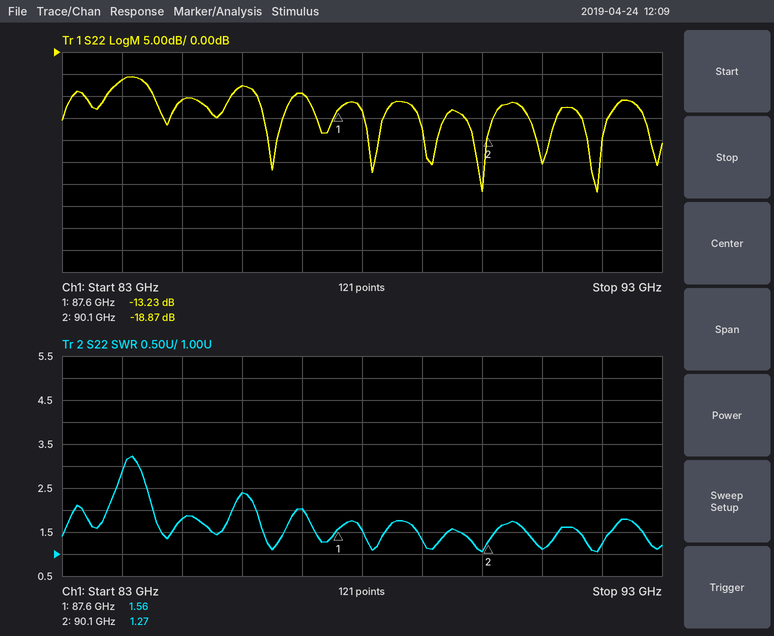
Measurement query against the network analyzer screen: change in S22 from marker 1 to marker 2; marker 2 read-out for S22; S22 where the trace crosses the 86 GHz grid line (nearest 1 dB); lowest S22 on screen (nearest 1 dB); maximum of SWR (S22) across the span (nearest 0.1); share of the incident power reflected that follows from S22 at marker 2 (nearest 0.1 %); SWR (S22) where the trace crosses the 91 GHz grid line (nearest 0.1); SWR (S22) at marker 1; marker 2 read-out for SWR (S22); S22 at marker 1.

-5.64 dB
-18.87 dB
-8 dB
-32 dB
3.2
1.3 %
1.1
1.56
1.27
-13.23 dB
